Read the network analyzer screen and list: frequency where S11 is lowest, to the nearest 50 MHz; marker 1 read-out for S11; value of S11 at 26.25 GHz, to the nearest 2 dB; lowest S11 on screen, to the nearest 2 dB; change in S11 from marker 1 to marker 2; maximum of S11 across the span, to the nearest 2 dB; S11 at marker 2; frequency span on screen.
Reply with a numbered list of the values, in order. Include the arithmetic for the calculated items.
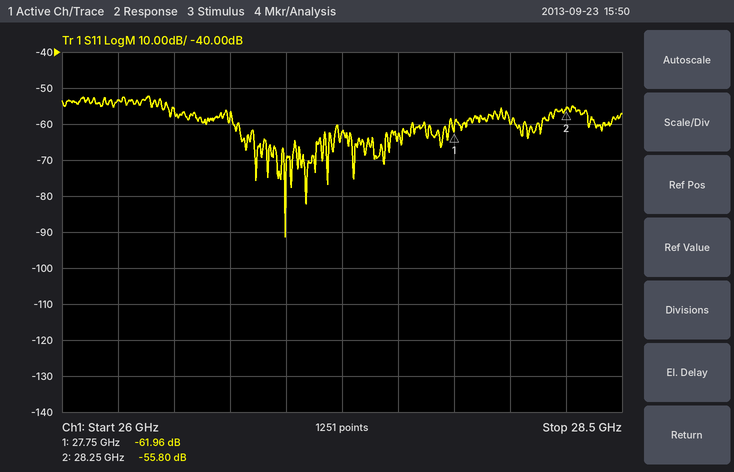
1. 27.00 GHz
2. -61.96 dB
3. -54 dB
4. -92 dB
5. -55.8 − (-61.96) = 6.16 dB
6. -52 dB
7. -55.80 dB
8. 2.5 GHz
